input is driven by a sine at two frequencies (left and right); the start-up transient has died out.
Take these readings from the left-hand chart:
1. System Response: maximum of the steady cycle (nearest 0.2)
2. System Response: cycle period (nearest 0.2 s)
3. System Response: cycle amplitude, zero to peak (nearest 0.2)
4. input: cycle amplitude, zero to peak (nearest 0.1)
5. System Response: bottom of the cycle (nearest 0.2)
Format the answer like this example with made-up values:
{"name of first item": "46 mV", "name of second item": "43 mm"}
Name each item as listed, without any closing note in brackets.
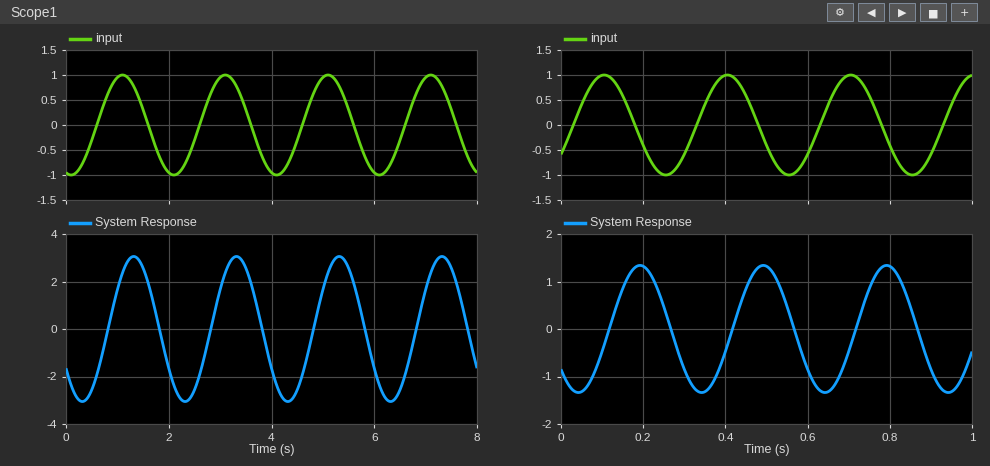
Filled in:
{"System Response: maximum of the steady cycle": "3.0", "System Response: cycle period": "2.0 s", "System Response: cycle amplitude, zero to peak": "3.0", "input: cycle amplitude, zero to peak": "1.0", "System Response: bottom of the cycle": "-3.0"}
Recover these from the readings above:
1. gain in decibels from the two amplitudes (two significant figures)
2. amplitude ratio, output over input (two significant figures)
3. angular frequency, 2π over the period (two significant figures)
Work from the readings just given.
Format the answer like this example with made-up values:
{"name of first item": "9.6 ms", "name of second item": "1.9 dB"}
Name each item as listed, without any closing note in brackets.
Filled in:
{"gain in decibels from the two amplitudes": "9.5 dB", "amplitude ratio, output over input": "3.0", "angular frequency, 2π over the period": "3.1 rad/s"}
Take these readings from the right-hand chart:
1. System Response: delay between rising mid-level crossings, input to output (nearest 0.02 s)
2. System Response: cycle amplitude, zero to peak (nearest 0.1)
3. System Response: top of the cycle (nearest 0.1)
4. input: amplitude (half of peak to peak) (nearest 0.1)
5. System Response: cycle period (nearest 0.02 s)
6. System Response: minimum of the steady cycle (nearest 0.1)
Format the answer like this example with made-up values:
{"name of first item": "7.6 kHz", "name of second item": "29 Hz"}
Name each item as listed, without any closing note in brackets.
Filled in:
{"System Response: delay between rising mid-level crossings, input to output": "0.08 s", "System Response: cycle amplitude, zero to peak": "1.3", "System Response: top of the cycle": "1.3", "input: amplitude (half of peak to peak)": "1.0", "System Response: cycle period": "0.30 s", "System Response: minimum of the steady cycle": "-1.3"}
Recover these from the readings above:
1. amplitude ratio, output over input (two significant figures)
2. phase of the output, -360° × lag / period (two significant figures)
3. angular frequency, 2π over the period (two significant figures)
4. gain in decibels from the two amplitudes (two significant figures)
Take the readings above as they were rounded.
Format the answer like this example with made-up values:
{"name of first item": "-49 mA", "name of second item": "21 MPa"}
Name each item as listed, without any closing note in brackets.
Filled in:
{"amplitude ratio, output over input": "1.3", "phase of the output, -360° × lag / period": "-96°", "angular frequency, 2π over the period": "21 rad/s", "gain in decibels from the two amplitudes": "2.3 dB"}
